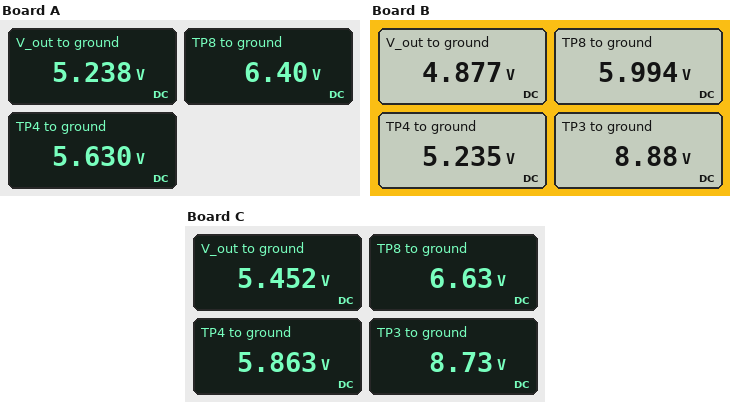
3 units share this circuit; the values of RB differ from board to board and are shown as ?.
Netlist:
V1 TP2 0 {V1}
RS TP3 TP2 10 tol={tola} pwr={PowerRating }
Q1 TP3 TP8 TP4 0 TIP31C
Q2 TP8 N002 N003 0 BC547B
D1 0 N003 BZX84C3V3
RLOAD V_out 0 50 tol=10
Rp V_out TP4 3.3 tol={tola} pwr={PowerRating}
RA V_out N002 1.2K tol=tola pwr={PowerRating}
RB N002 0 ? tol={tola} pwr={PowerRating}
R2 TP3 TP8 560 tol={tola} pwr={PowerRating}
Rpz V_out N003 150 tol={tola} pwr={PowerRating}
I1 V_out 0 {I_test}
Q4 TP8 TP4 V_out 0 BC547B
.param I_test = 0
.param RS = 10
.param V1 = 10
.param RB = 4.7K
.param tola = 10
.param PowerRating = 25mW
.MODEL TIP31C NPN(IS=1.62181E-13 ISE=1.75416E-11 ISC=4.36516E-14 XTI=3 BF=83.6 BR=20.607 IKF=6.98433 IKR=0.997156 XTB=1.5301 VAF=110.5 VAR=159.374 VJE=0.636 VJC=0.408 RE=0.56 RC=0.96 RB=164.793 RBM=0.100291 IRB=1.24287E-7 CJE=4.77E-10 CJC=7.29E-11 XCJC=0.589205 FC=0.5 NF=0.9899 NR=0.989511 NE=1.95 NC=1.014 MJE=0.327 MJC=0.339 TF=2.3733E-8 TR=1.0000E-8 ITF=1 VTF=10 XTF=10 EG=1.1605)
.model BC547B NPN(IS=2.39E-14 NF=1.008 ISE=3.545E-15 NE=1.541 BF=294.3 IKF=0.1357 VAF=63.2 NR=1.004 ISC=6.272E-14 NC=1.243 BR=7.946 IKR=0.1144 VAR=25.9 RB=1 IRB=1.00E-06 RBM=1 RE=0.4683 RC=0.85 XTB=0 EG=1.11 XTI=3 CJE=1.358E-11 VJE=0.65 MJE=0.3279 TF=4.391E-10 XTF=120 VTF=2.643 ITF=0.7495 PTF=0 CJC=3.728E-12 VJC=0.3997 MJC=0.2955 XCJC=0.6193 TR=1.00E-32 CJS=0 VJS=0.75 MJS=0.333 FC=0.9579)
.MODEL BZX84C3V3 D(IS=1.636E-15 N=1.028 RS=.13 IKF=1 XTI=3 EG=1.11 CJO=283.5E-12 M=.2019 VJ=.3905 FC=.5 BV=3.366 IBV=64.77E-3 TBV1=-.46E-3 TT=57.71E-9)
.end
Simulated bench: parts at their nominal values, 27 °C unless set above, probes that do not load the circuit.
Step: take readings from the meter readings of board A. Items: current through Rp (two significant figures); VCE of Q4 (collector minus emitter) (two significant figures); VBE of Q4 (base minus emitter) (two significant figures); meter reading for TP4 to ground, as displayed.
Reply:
120 mA
1.2 V
390 mV
5.630 V
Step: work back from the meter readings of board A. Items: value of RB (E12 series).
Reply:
3.9 kΩ
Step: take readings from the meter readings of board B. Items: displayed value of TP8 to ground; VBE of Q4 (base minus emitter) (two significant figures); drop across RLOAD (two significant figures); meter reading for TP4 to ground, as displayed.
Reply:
5.994 V
360 mV
4.9 V
5.235 V
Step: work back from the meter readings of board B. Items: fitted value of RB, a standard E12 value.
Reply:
5.6 kΩ
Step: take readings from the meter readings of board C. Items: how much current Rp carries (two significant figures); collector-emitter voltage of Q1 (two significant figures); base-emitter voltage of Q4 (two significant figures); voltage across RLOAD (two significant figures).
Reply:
120 mA
2.9 V
410 mV
5.5 V
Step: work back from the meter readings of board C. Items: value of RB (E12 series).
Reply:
3.3 kΩ
